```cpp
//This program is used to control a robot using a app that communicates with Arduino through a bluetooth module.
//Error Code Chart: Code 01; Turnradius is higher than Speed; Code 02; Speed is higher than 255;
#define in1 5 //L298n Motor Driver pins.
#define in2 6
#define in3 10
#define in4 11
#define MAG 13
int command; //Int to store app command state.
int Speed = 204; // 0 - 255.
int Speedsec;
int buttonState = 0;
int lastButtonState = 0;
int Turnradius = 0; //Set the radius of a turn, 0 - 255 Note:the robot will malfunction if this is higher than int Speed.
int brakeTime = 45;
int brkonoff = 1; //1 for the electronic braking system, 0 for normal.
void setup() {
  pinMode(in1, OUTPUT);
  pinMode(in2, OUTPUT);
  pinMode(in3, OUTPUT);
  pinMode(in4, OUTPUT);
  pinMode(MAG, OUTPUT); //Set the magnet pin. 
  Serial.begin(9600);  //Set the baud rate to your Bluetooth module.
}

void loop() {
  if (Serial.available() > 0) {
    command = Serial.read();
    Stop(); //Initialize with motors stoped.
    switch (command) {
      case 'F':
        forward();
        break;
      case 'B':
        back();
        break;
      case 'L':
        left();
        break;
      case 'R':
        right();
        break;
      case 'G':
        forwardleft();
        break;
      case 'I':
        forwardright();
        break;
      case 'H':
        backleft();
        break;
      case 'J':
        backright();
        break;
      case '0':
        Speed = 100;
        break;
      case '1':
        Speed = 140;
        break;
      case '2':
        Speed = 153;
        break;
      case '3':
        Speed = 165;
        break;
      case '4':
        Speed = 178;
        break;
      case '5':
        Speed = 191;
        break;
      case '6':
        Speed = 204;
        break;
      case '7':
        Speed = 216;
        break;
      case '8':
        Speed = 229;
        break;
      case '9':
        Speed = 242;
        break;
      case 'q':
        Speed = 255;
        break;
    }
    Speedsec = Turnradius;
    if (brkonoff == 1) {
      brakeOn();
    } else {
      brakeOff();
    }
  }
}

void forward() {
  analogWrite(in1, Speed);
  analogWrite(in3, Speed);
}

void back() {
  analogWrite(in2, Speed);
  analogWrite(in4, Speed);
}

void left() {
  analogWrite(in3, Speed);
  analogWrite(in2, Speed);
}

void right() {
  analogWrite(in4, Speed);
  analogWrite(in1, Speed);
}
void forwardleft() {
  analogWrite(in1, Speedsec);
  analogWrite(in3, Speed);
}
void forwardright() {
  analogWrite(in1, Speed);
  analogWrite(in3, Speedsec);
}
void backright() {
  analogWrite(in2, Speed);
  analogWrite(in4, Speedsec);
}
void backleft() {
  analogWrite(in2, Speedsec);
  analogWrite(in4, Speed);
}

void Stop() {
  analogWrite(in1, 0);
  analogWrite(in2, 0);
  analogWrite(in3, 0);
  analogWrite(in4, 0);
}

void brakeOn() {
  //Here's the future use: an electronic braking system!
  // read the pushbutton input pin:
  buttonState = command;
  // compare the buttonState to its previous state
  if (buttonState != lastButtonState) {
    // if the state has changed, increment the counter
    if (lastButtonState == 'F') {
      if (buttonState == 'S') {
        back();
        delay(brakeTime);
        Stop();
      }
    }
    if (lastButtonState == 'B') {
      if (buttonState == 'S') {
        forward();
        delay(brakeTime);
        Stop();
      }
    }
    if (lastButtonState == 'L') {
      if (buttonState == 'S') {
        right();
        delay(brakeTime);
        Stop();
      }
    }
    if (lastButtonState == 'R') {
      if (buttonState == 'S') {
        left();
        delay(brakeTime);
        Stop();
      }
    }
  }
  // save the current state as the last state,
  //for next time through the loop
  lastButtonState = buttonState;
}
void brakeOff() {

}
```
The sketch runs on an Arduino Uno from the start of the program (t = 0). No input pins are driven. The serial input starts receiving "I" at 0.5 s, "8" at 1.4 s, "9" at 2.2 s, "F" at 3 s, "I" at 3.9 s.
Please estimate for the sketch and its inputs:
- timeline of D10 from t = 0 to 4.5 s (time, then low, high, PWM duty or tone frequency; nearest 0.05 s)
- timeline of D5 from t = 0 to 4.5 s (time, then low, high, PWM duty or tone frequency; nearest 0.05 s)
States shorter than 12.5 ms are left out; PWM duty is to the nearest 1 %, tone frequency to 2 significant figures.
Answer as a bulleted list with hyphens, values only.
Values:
- 0 s low; 3 s PWM 95 %; 3.9 s low
- 0 s low; 0.5 s PWM 80 %; 1.4 s low; 3 s PWM 95 %
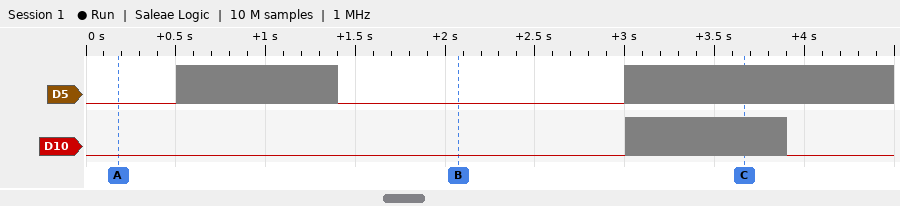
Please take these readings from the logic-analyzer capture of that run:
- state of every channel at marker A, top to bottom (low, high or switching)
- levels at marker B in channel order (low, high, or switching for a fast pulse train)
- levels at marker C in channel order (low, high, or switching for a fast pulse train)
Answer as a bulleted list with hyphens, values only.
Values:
- D5 low, D10 low
- D5 low, D10 low
- D5 switching, D10 switching
